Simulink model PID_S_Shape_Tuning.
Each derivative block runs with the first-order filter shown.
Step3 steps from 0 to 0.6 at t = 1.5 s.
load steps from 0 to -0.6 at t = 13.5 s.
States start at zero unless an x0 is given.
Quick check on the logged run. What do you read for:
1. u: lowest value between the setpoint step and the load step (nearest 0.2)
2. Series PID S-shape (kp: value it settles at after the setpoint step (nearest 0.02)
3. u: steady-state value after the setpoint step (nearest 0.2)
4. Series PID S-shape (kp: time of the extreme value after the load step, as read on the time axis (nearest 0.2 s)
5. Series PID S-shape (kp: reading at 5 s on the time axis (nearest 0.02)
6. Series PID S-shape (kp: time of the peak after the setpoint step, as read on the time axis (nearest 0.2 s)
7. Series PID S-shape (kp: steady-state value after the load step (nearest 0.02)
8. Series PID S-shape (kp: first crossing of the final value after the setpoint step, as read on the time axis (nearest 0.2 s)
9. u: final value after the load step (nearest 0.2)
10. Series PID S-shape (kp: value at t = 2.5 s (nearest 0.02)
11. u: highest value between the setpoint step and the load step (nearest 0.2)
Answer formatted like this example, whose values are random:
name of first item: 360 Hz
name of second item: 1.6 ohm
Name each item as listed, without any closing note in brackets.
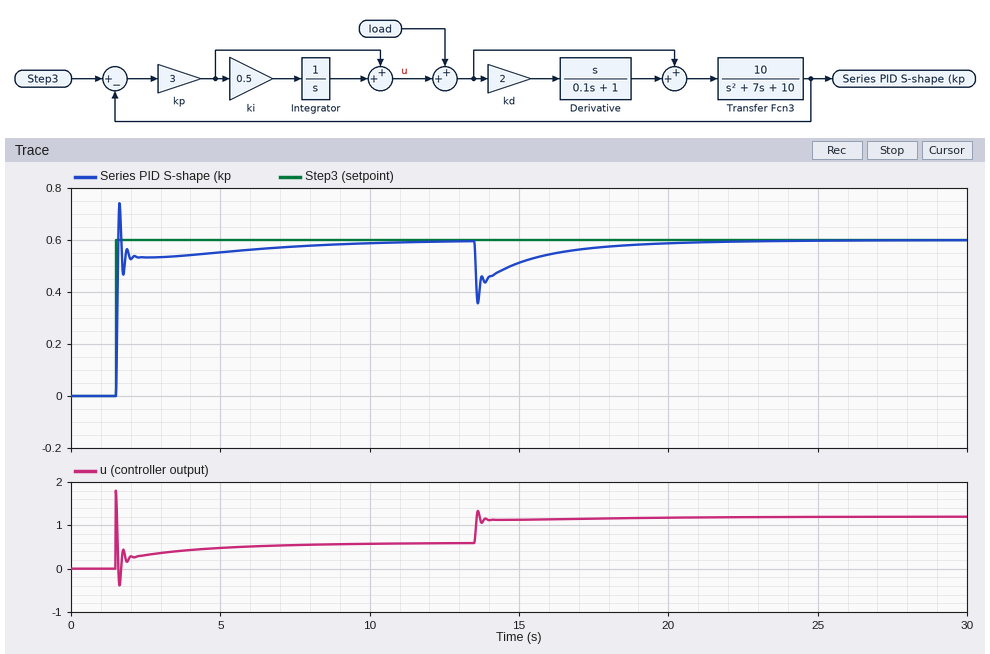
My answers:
u: lowest value between the setpoint step and the load step: -0.4
Series PID S-shape (kp: value it settles at after the setpoint step: 0.60
u: steady-state value after the setpoint step: 0.6
Series PID S-shape (kp: time of the extreme value after the load step, as read on the time axis: 13.6 s
Series PID S-shape (kp: reading at 5 s on the time axis: 0.56
Series PID S-shape (kp: time of the peak after the setpoint step, as read on the time axis: 1.6 s
Series PID S-shape (kp: steady-state value after the load step: 0.60
Series PID S-shape (kp: first crossing of the final value after the setpoint step, as read on the time axis: 1.6 s
u: final value after the load step: 1.2
Series PID S-shape (kp: value at t = 2.5 s: 0.54
u: highest value between the setpoint step and the load step: 1.8
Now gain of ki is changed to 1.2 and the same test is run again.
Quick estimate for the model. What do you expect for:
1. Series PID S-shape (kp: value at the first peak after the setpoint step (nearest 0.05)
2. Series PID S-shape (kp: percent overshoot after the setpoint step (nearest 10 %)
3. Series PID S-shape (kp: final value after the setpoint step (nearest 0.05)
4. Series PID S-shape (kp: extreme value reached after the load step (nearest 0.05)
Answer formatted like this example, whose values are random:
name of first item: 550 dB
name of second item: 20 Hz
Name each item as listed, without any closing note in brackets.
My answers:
Series PID S-shape (kp: value at the first peak after the setpoint step: 0.75
Series PID S-shape (kp: percent overshoot after the setpoint step: 30 %
Series PID S-shape (kp: final value after the setpoint step: 0.60
Series PID S-shape (kp: extreme value reached after the load step: 0.35
